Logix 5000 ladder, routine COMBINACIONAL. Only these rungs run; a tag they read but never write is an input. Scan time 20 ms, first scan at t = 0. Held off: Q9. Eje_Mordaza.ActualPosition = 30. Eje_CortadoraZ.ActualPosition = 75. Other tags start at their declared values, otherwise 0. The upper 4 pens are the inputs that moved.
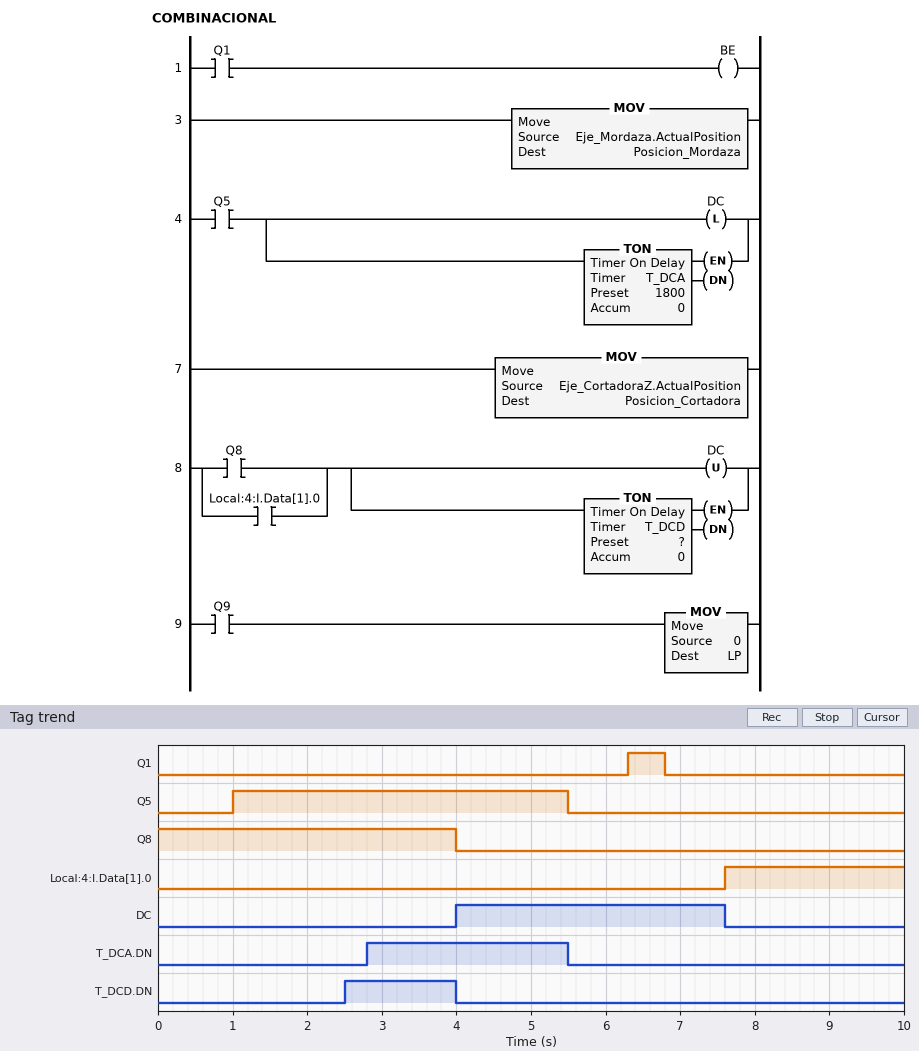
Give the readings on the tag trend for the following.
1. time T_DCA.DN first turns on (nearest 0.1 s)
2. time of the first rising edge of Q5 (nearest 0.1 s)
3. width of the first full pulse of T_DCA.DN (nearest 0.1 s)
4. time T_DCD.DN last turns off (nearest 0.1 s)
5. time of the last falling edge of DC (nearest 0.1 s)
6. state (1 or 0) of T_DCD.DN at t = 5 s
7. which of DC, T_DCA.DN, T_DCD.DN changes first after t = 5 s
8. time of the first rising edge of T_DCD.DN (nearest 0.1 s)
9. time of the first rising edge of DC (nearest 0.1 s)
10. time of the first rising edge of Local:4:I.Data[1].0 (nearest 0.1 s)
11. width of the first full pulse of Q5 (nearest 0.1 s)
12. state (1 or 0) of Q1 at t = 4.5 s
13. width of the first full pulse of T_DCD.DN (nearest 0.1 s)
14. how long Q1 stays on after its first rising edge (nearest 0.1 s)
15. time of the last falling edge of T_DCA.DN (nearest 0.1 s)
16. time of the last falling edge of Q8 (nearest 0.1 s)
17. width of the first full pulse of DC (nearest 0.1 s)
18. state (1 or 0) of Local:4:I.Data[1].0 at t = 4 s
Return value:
2.8 s
1.0 s
2.7 s
4.0 s
7.6 s
0
T_DCA.DN
2.5 s
4.0 s
7.6 s
4.5 s
0
1.5 s
0.5 s
5.5 s
4.0 s
3.6 s
0
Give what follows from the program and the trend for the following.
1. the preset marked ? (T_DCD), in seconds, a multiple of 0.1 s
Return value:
2.5 s
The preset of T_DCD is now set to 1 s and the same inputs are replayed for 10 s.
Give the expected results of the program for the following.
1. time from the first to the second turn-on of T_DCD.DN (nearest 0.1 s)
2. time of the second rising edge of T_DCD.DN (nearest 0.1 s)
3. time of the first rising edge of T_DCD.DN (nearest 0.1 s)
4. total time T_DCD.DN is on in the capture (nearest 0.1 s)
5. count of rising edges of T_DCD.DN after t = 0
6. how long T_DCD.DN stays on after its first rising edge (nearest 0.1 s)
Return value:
7.6 s
8.6 s
1.0 s
4.4 s
2
3.0 s
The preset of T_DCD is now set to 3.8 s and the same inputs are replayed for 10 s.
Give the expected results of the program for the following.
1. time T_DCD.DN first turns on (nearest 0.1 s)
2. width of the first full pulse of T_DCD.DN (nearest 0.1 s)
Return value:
3.8 s
0.2 s
